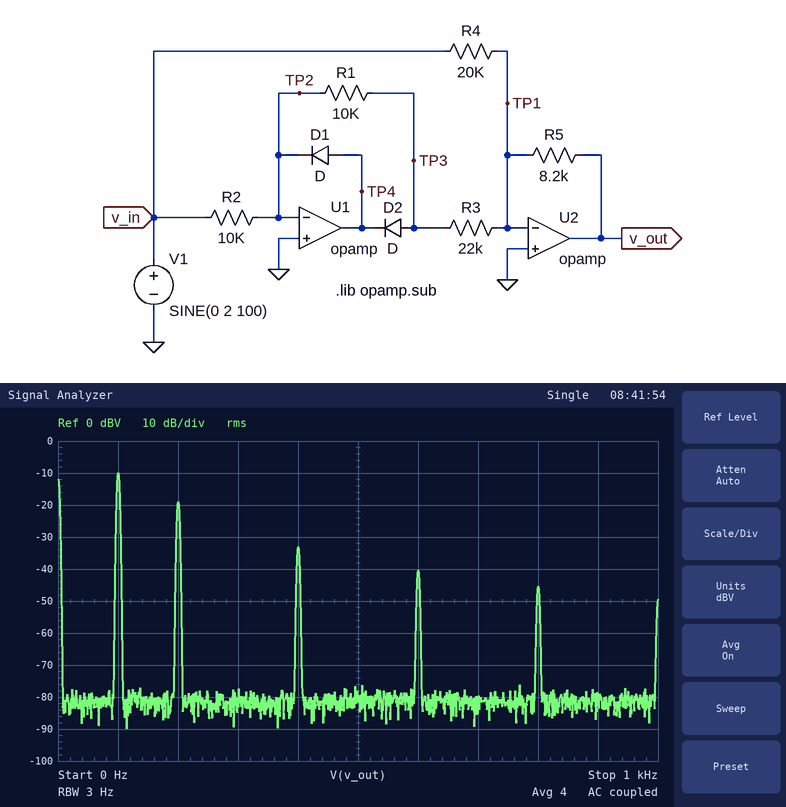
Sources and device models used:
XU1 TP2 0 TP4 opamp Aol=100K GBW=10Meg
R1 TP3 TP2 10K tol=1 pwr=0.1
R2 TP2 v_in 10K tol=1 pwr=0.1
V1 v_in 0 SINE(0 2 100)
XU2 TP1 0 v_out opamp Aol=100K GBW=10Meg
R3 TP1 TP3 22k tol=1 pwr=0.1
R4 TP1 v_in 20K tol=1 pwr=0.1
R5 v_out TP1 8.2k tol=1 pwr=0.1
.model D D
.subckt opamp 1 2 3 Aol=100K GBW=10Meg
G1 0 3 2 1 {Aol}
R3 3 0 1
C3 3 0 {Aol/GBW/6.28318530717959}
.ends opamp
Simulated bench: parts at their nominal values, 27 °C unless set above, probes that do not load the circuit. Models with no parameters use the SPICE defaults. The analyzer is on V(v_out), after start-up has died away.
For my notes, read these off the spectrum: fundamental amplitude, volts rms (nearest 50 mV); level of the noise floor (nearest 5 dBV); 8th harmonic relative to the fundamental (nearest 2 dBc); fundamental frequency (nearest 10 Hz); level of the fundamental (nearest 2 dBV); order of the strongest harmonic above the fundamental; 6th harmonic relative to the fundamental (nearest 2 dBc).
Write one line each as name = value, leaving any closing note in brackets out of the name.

fundamental amplitude, volts rms = 300 mV
level of the noise floor = -80 dBV
8th harmonic relative to the fundamental = -36 dBc
fundamental frequency = 100 Hz
level of the fundamental = -10 dBV
order of the strongest harmonic above the fundamental = 2
6th harmonic relative to the fundamental = -30 dBc
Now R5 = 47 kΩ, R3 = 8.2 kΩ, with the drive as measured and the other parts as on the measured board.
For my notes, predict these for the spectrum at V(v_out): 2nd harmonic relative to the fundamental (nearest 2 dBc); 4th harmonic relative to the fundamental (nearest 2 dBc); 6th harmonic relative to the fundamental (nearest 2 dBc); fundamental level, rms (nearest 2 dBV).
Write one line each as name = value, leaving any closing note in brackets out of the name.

2nd harmonic relative to the fundamental = 8 dBc
4th harmonic relative to the fundamental = -6 dBc
6th harmonic relative to the fundamental = -14 dBc
fundamental level, rms = -2 dBV
